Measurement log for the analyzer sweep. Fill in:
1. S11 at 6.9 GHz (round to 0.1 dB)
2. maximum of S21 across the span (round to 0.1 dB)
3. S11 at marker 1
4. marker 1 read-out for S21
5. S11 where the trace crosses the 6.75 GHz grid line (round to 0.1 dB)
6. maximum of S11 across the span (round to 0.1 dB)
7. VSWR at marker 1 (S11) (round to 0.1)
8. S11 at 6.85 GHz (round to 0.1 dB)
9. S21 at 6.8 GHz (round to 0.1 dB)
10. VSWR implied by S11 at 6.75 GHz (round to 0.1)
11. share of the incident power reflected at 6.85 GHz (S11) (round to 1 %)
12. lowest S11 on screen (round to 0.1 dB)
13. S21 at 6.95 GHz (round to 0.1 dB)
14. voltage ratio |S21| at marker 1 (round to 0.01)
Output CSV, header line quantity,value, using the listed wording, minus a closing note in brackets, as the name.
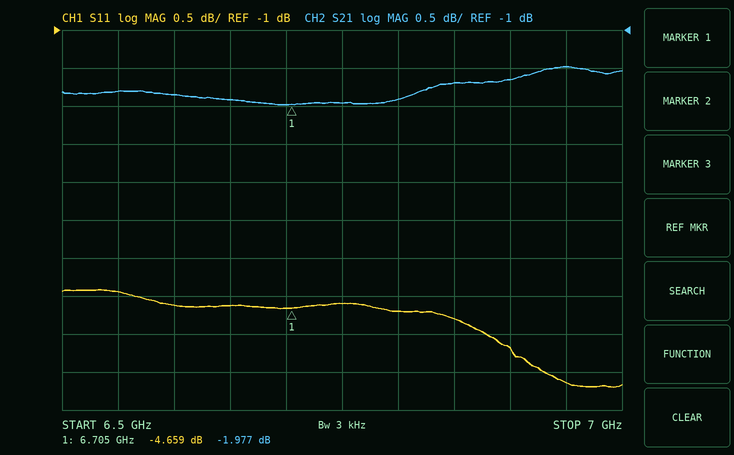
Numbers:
quantity,value
S11 at 6.9 GHz,-5.2 dB
maximum of S21 across the span,-1.5 dB
S11 at marker 1,-4.659 dB
marker 1 read-out for S21,-1.977 dB
S11 where the trace crosses the 6.75 GHz grid line,-4.6 dB
maximum of S11 across the span,-4.4 dB
VSWR at marker 1 (S11),3.8
S11 at 6.85 GHz,-4.8 dB
S21 at 6.8 GHz,-1.9 dB
VSWR implied by S11 at 6.75 GHz,3.9
share of the incident power reflected at 6.85 GHz (S11),33 %
lowest S11 on screen,-5.7 dB
S21 at 6.95 GHz,-1.5 dB
voltage ratio |S21| at marker 1,0.80
